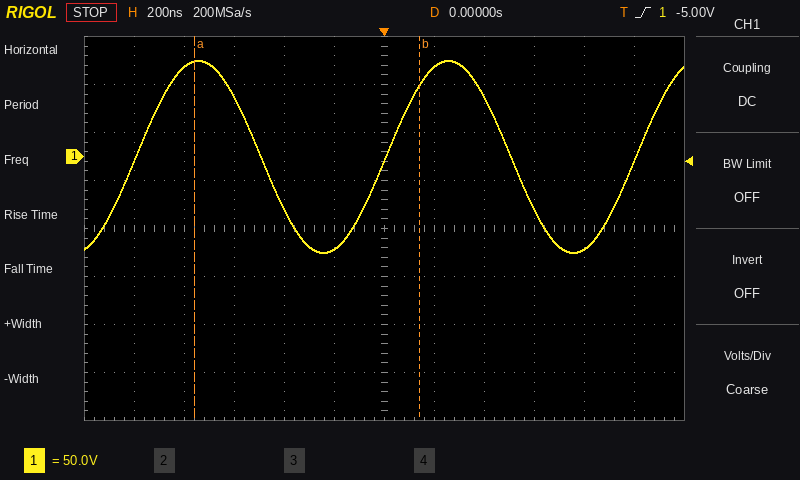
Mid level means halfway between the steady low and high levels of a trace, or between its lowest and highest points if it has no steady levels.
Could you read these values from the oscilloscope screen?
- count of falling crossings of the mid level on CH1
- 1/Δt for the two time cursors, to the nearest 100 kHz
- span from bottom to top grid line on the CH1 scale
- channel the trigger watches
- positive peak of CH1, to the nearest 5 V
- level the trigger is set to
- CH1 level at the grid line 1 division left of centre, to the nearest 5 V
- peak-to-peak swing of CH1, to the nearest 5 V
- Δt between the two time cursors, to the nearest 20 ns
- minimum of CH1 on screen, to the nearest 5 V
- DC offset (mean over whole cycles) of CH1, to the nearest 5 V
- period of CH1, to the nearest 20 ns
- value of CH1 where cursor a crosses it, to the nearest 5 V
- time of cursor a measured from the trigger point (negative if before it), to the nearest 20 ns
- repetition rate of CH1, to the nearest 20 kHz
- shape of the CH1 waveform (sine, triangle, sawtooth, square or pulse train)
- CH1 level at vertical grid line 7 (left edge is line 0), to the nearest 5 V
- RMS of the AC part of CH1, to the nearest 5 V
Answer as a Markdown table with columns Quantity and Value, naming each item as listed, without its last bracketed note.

| Quantity | Value |
|---|---|
| count of falling crossings of the mid level on CH1 | 2 |
| 1/Δt for the two time cursors, to the nearest 100 kHz | 1.1 MHz |
| span from bottom to top grid line on the CH1 scale | 400 V |
| channel the trigger watches | CH1 |
| positive peak of CH1, to the nearest 5 V | 100 V |
| level the trigger is set to | -5.00 V |
| CH1 level at the grid line 1 division left of centre, to the nearest 5 V | -95 V |
| peak-to-peak swing of CH1, to the nearest 5 V | 200 V |
| Δt between the two time cursors, to the nearest 20 ns | 900 ns |
| minimum of CH1 on screen, to the nearest 5 V | -100 V |
| DC offset (mean over whole cycles) of CH1, to the nearest 5 V | 0 V |
| period of CH1, to the nearest 20 ns | 1.00 µs |
| value of CH1 where cursor a crosses it, to the nearest 5 V | 100 V |
| time of cursor a measured from the trigger point (negative if before it), to the nearest 20 ns | -760 ns |
| repetition rate of CH1, to the nearest 20 kHz | 1.00 MHz |
| shape of the CH1 waveform | sine |
| CH1 level at vertical grid line 7 (left edge is line 0), to the nearest 5 V | 95 V |
| RMS of the AC part of CH1, to the nearest 5 V | 70 V |
